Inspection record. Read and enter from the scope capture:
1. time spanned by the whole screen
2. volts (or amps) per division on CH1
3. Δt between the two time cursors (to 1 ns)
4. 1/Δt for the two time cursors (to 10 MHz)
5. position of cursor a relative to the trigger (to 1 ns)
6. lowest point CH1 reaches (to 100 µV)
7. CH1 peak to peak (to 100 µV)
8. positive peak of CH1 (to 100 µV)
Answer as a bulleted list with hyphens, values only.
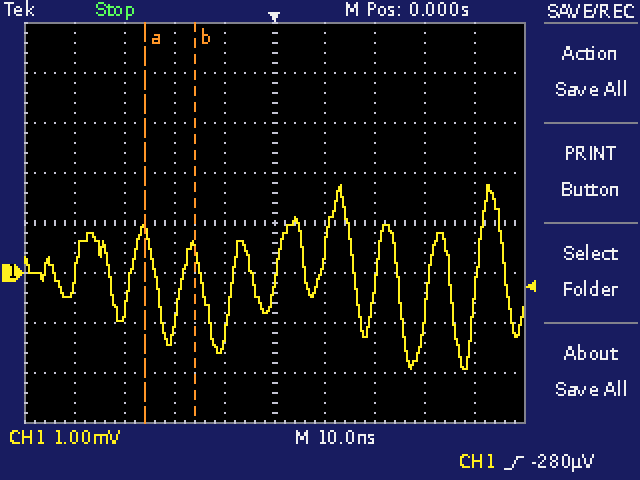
- 100 ns
- 1 mV
- 10 ns
- 100 MHz
- -26 ns
- -1.9 mV
- 3.7 mV
- 1.8 mV
